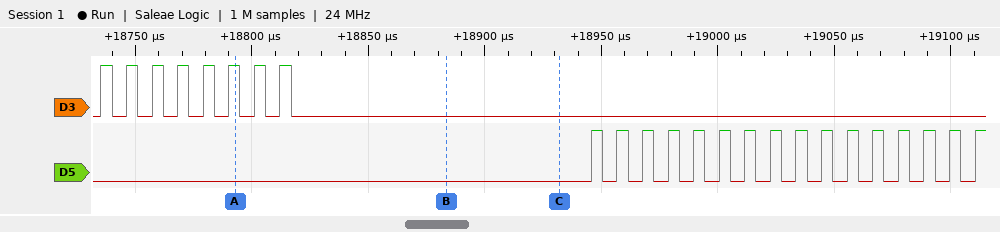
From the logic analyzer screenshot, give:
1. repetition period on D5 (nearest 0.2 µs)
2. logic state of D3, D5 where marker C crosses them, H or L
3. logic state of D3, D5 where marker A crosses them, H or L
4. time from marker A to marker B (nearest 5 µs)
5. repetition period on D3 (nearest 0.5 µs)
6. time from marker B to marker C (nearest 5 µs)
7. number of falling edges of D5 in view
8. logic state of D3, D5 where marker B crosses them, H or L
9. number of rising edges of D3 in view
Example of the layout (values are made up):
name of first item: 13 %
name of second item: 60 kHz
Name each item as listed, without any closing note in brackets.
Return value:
repetition period on D5: 11 µs
logic state of D3, D5 where marker C crosses them, H or L: D3=L, D5=L
logic state of D3, D5 where marker A crosses them, H or L: D3=H, D5=L
time from marker A to marker B: 90 µs
repetition period on D3: 11 µs
time from marker B to marker C: 50 µs
number of falling edges of D5 in view: 15
logic state of D3, D5 where marker B crosses them, H or L: D3=L, D5=L
number of rising edges of D3 in view: 8
